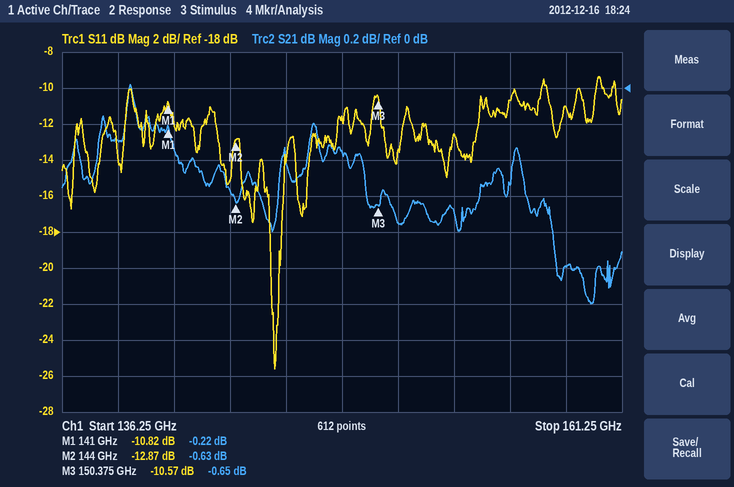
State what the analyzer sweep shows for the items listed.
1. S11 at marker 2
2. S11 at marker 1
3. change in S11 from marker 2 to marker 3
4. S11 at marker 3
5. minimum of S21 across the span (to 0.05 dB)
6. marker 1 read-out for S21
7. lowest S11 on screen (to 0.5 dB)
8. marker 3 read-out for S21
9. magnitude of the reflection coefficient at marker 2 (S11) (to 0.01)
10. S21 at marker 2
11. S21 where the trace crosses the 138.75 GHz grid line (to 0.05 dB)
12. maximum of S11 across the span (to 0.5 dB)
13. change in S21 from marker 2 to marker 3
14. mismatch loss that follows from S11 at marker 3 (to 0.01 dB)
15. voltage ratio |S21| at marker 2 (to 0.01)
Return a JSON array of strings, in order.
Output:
["-12.87 dB", "-10.82 dB", "2.30 dB", "-10.57 dB", "-1.20 dB", "-0.22 dB", "-25.5 dB", "-0.65 dB", "0.23", "-0.63 dB", "-0.30 dB", "-9.5 dB", "-0.02 dB", "0.40 dB", "0.93"]
